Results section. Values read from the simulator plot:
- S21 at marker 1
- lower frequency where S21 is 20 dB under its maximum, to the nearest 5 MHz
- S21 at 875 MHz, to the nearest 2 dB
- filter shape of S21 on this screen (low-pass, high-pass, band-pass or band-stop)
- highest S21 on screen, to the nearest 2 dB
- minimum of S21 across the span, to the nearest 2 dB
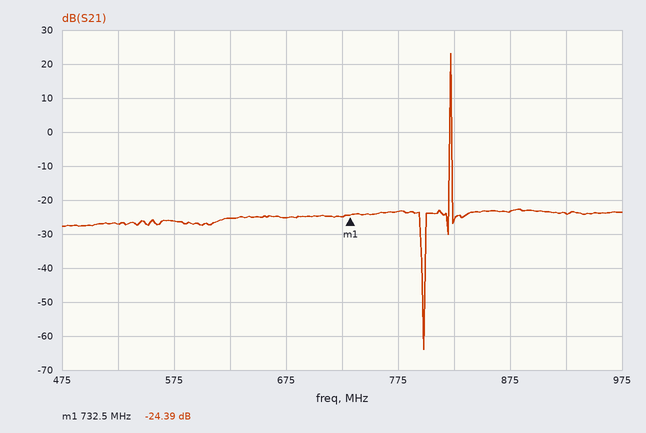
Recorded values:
-24.39 dB
820 MHz
-24 dB
band-pass
24 dB
-64 dB
